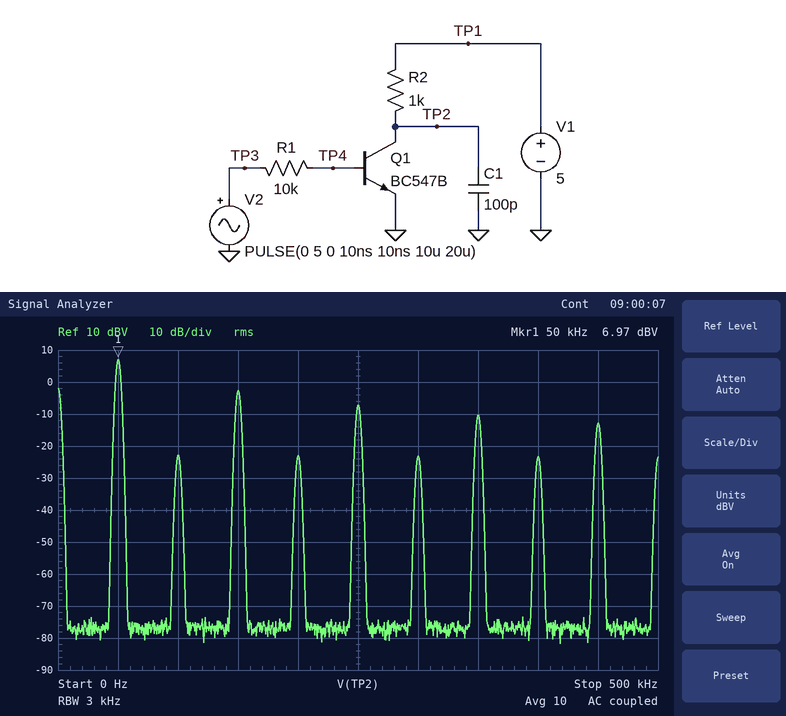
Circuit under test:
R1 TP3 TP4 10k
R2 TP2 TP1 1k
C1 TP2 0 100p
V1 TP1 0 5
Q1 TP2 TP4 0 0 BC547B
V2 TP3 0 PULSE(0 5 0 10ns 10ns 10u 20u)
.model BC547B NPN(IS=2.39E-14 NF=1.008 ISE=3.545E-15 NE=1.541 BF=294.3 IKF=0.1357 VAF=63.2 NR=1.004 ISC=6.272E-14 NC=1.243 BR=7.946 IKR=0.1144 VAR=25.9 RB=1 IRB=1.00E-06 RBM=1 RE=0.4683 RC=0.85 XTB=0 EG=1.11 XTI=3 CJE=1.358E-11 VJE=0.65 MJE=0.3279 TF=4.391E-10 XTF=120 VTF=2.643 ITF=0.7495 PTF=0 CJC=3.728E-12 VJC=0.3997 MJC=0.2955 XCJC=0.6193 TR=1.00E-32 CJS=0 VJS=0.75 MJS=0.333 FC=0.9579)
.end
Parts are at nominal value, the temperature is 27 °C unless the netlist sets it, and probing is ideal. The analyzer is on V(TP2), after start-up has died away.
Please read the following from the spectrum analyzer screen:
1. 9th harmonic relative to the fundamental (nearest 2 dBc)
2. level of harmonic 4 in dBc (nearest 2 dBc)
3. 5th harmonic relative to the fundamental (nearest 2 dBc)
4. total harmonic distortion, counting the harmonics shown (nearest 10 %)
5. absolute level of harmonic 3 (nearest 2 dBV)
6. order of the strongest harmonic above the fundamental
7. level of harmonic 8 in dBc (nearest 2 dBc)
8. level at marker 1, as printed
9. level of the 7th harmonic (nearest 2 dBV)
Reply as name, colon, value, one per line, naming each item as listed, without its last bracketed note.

9th harmonic relative to the fundamental: -20 dBc
level of harmonic 4 in dBc: -30 dBc
5th harmonic relative to the fundamental: -14 dBc
total harmonic distortion, counting the harmonics shown: 40 %
absolute level of harmonic 3: -2 dBV
order of the strongest harmonic above the fundamental: 3
level of harmonic 8 in dBc: -30 dBc
level at marker 1, as printed: 6.97 dBV
level of the 7th harmonic: -10 dBV
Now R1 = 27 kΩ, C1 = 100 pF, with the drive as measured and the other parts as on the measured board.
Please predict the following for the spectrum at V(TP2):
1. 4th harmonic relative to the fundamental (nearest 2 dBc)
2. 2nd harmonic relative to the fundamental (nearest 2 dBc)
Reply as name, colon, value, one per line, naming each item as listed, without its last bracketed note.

4th harmonic relative to the fundamental: -26 dBc
2nd harmonic relative to the fundamental: -26 dBc
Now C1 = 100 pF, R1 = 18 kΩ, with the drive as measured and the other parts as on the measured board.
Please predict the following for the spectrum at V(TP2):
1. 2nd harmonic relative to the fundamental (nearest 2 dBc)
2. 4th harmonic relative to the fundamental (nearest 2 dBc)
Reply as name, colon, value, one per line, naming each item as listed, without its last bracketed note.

2nd harmonic relative to the fundamental: -28 dBc
4th harmonic relative to the fundamental: -28 dBc
